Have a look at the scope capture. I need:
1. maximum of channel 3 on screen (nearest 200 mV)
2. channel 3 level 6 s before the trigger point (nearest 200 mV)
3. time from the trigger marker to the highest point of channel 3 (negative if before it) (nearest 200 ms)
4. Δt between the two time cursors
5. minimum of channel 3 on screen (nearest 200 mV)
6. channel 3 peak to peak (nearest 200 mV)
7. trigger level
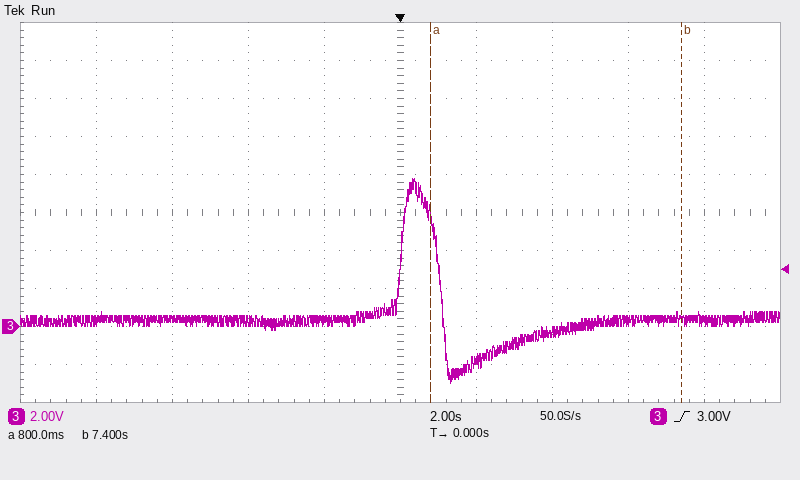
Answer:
7.8 V
400 mV
+400 ms
6.6 s
-3.0 V
10.8 V
3.00 V
